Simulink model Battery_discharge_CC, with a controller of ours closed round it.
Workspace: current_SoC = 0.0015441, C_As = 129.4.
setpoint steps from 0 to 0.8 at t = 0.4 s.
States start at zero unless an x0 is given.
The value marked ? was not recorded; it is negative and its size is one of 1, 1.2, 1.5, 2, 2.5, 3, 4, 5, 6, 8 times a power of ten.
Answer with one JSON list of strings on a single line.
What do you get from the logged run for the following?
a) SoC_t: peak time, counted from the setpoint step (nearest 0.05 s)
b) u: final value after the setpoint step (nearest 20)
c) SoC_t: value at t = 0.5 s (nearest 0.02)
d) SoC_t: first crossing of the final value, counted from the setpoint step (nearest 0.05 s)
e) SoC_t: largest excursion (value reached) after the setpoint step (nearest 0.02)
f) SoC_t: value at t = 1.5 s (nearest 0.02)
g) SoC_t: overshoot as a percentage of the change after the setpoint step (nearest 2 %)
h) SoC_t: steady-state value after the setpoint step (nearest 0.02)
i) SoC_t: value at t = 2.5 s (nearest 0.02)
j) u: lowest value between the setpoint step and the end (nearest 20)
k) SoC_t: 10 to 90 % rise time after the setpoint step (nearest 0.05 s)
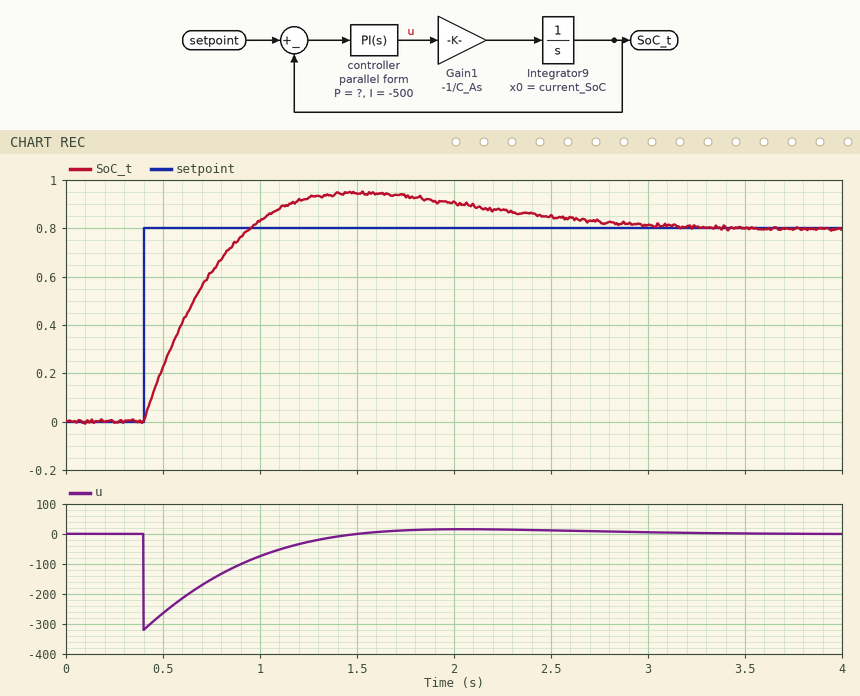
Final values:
["1.10 s", "0", "0.22", "0.55 s", "0.94", "0.94", "18 %", "0.80", "0.84", "-320", "0.40 s"]
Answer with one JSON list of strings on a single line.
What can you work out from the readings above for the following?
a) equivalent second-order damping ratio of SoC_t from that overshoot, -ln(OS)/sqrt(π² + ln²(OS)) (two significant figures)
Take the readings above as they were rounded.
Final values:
["0.48"]
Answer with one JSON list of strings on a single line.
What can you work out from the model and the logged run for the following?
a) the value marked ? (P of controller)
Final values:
["-400"]
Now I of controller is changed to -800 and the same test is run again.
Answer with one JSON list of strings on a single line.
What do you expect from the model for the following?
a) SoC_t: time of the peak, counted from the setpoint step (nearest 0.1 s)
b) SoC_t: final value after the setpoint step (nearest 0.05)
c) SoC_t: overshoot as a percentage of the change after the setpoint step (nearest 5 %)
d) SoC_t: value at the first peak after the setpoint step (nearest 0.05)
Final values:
["0.9 s", "0.80", "25 %", "1.00"]
